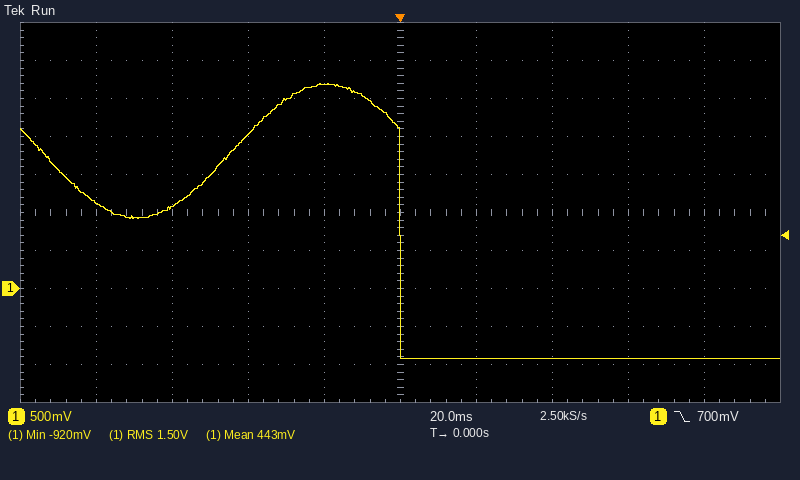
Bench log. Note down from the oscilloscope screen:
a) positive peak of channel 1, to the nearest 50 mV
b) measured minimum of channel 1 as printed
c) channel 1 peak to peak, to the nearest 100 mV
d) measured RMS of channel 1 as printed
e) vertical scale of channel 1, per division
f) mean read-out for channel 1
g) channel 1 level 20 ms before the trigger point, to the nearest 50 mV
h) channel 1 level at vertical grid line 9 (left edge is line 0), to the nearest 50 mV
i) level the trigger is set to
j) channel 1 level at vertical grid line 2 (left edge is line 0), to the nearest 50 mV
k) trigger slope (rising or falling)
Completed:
2.70 V
-920 mV
3.60 V
1.50 V
500 mV
443 mV
2.70 V
-900 mV
700 mV
1.10 V
falling
